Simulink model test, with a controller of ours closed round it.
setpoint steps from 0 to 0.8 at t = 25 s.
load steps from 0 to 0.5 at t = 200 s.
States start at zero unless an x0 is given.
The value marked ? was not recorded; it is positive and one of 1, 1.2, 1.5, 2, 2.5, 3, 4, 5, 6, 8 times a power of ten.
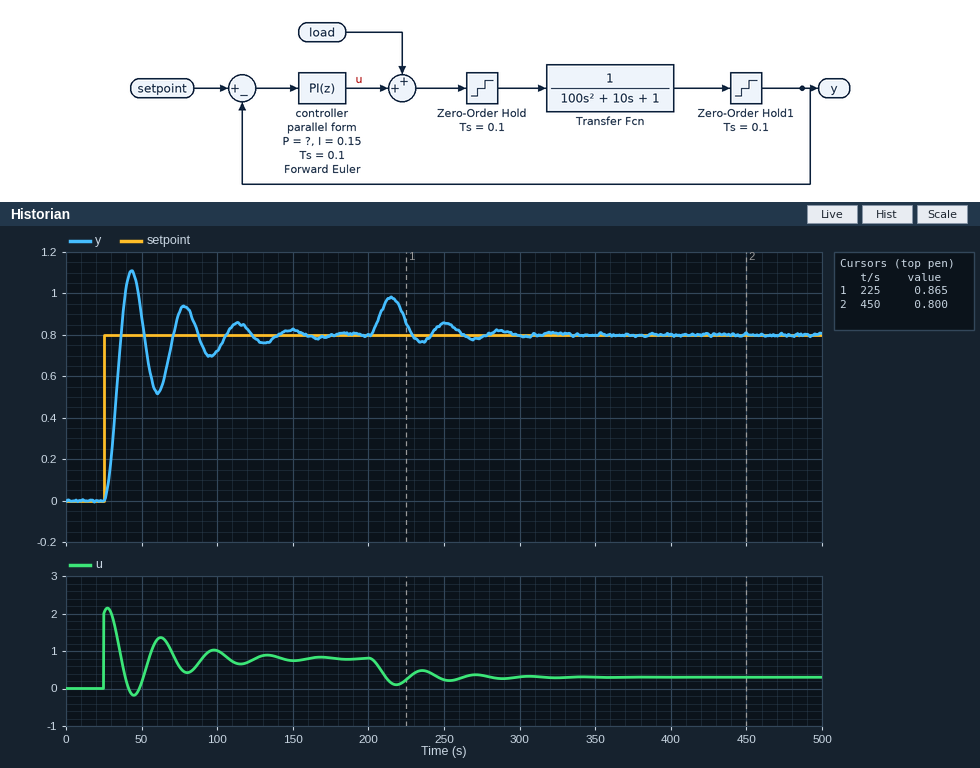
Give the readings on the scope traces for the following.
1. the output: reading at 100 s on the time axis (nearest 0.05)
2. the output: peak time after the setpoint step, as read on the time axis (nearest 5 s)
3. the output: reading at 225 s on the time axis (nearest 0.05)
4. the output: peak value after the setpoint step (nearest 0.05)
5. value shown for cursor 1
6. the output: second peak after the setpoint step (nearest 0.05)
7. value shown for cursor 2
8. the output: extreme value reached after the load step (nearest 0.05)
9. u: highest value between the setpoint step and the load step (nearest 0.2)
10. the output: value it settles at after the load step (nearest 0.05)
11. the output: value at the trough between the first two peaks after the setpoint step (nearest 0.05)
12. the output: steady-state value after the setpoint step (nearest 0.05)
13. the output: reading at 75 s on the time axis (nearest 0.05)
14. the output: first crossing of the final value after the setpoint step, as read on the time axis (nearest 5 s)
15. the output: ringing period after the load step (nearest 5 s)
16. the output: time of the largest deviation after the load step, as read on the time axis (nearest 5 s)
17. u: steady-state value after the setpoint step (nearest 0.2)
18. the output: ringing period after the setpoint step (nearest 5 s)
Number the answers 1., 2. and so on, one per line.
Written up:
1. 0.70
2. 45 s
3. 0.85
4. 1.10
5. 0.865
6. 0.95
7. 0.800
8. 1.00
9. 2.2
10. 0.80
11. 0.50
12. 0.80
13. 0.90
14. 35 s
15. 35 s
16. 215 s
17. 0.8
18. 35 s
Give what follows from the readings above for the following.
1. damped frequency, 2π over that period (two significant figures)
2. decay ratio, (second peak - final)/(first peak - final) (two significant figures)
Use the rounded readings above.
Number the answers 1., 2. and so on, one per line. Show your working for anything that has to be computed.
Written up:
1. 2π / 35 = 0.18 rad/s
2. (0.95 - 0.8) / (1.1 - 0.8) = 0.50
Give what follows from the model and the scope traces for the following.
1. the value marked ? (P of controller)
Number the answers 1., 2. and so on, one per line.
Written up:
1. 2.5
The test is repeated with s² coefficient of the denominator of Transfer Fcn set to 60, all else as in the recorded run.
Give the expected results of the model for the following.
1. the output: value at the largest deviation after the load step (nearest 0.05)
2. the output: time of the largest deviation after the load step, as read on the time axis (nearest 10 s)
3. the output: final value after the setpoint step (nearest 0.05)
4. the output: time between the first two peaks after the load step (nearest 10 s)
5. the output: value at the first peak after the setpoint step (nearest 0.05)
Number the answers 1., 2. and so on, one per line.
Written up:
1. 0.95
2. 210 s
3. 0.80
4. 30 s
5. 1.00
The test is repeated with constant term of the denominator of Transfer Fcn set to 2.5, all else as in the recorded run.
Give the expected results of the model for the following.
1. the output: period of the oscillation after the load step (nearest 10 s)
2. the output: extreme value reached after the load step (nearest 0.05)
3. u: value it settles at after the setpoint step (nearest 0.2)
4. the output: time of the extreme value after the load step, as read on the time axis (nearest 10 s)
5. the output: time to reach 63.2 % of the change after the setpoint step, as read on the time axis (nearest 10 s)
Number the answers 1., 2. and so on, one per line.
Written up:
1. 30 s
2. 0.95
3. 2.0
4. 210 s
5. 30 s
